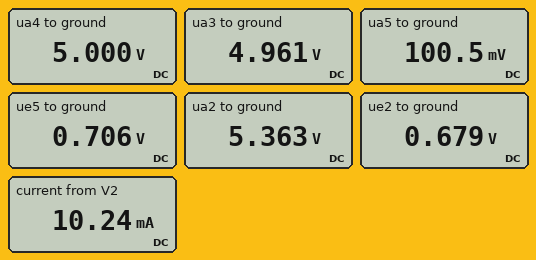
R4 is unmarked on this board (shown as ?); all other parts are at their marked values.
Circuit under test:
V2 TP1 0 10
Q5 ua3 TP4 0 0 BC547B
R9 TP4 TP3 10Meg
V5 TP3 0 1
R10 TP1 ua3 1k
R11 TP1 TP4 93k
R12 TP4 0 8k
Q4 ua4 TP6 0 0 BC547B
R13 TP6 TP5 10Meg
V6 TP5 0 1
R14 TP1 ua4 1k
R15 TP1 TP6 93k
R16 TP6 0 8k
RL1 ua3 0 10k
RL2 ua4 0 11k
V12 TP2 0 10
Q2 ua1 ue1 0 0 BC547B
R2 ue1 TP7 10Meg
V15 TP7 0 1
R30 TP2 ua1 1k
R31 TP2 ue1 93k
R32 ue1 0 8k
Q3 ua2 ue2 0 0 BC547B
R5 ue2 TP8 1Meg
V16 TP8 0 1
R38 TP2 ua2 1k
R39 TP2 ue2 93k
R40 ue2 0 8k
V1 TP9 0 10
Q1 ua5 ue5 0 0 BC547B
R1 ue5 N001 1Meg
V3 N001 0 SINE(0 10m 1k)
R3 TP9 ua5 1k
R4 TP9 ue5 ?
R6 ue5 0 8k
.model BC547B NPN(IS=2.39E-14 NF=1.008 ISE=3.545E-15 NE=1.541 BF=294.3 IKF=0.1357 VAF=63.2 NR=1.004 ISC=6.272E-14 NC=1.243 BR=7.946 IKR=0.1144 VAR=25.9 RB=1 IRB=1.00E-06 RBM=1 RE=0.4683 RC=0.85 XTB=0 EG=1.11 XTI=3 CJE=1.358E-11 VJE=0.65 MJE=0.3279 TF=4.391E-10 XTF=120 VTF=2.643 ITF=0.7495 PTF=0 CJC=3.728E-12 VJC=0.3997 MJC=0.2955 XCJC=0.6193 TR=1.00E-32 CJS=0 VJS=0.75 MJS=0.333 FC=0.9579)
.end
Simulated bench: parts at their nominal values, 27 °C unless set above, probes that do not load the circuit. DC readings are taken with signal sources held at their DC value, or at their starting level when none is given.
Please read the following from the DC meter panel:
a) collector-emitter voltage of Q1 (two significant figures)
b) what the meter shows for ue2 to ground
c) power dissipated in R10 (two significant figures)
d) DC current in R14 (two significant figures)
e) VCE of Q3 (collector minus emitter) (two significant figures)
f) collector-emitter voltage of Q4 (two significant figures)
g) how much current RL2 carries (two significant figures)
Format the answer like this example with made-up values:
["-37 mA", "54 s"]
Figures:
["100 mV", "0.679 V", "25 mW", "5.0 mA", "5.4 V", "5.0 V", "450 µA"]
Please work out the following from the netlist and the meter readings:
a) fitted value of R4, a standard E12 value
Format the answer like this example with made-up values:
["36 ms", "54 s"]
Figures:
["47 kΩ"]
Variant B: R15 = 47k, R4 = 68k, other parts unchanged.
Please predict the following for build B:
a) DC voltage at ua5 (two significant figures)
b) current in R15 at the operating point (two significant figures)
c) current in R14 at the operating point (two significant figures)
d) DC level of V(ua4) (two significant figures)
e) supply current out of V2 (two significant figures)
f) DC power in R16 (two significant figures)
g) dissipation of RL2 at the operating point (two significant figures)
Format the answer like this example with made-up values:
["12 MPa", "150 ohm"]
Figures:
["150 mV", "200 µA", "9.9 mA", "100 mV", "15 mA", "62 µW", "910 nW"]
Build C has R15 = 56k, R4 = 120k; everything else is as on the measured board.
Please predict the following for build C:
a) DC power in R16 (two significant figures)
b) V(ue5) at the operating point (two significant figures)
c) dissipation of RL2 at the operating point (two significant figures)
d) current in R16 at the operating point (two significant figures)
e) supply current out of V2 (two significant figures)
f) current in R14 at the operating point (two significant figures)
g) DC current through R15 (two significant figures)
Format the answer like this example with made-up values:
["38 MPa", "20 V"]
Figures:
["62 µW", "610 mV", "1.2 µW", "88 µA", "15 mA", "9.9 mA", "170 µA"]
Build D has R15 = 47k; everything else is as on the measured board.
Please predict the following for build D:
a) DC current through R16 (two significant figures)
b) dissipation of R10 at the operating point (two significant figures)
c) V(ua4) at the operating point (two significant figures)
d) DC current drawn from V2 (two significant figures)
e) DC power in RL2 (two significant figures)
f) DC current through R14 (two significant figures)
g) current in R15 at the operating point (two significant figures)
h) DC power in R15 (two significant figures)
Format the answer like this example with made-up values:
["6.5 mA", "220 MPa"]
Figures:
["88 µA", "25 mW", "100 mV", "15 mA", "910 nW", "9.9 mA", "200 µA", "1.8 mW"]
